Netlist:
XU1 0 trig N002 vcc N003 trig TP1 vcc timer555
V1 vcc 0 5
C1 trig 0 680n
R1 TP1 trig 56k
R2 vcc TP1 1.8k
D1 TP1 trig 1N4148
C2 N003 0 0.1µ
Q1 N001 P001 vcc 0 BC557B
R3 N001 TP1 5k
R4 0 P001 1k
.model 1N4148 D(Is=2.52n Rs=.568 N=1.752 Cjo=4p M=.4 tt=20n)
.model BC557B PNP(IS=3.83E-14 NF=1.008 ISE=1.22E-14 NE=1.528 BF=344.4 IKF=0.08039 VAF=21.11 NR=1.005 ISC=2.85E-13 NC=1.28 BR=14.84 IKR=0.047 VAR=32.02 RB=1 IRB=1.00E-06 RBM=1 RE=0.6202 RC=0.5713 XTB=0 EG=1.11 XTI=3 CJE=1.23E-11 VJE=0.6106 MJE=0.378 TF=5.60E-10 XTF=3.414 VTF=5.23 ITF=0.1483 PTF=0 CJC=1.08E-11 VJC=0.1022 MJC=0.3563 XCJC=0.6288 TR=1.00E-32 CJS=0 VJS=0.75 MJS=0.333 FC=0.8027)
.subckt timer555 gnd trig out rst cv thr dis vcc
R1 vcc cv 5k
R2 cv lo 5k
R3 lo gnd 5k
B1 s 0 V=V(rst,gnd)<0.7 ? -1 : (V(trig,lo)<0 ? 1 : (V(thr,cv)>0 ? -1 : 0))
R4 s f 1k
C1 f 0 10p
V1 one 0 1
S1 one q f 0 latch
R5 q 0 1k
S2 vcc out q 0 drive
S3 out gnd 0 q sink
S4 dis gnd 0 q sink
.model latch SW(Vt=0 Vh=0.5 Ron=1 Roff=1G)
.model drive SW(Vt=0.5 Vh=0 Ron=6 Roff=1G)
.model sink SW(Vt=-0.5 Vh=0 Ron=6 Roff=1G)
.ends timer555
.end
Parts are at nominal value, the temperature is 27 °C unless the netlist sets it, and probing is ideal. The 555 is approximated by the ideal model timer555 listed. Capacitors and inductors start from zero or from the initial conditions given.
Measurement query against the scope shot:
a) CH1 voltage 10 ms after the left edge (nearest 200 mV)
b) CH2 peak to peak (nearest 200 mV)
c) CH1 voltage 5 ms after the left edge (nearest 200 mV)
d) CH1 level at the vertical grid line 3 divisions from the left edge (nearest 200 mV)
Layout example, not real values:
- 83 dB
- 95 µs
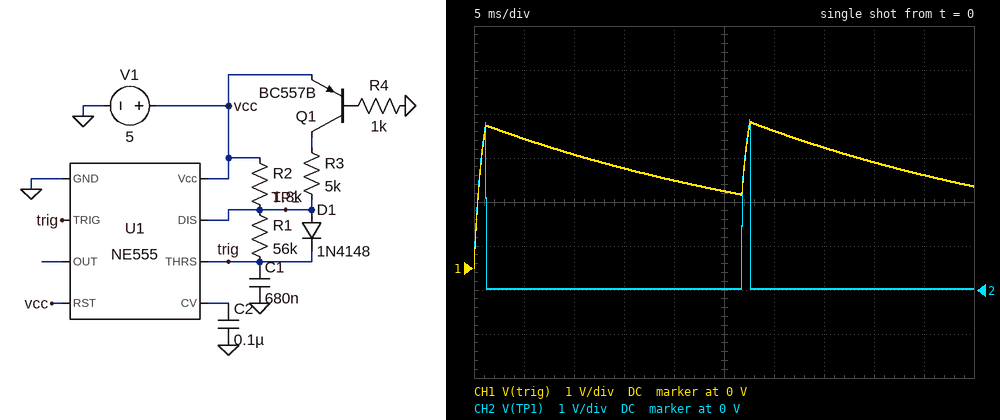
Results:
- 2.6 V
- 3.8 V
- 3.0 V
- 2.2 V
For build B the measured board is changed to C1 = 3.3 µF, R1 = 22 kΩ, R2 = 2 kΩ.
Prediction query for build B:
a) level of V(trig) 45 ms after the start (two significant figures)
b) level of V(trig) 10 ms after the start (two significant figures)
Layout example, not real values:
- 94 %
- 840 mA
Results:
- 2.0 V
- 3.2 V
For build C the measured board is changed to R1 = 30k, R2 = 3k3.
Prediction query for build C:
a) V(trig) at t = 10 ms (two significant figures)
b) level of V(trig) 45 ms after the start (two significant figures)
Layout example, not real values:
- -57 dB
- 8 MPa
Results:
- 2.2 V
- 1.8 V
